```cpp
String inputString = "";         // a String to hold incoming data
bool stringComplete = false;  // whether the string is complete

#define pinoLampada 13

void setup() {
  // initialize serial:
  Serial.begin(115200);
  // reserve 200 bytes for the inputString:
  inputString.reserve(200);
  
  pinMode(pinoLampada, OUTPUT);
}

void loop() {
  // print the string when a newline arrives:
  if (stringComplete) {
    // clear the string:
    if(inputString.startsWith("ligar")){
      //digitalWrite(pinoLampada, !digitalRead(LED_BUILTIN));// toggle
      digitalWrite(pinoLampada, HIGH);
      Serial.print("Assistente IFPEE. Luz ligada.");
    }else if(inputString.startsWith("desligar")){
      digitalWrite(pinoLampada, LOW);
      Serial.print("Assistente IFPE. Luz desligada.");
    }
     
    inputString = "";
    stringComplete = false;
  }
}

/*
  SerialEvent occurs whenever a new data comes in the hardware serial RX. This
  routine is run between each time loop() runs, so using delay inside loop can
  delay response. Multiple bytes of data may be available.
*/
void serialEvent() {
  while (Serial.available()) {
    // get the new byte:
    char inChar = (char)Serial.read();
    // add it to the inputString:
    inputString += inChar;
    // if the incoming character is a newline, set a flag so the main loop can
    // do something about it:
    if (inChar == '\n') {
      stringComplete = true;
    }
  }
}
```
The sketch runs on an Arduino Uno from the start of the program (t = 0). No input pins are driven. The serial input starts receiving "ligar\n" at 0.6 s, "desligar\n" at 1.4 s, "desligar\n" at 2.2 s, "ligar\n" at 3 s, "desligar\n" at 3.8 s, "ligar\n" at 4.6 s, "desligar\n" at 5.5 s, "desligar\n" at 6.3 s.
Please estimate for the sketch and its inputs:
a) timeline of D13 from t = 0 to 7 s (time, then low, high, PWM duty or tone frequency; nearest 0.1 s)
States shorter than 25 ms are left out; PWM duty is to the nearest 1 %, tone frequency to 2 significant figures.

0 s low; 0.6 s high; 1.4 s low; 3 s high; 3.8 s low; 4.6 s high; 5.5 s low
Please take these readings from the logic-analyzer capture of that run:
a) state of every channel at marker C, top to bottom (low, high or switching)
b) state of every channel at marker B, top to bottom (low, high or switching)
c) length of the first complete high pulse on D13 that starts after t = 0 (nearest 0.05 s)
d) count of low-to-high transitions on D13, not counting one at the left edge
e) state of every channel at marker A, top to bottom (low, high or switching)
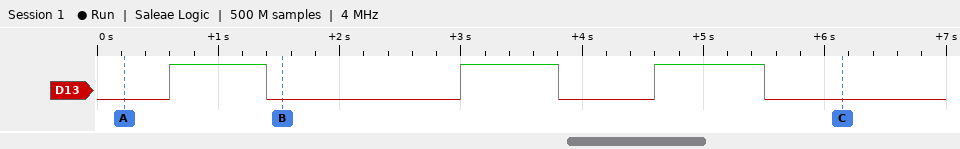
D13 low
D13 low
0.80 s
3
D13 low
